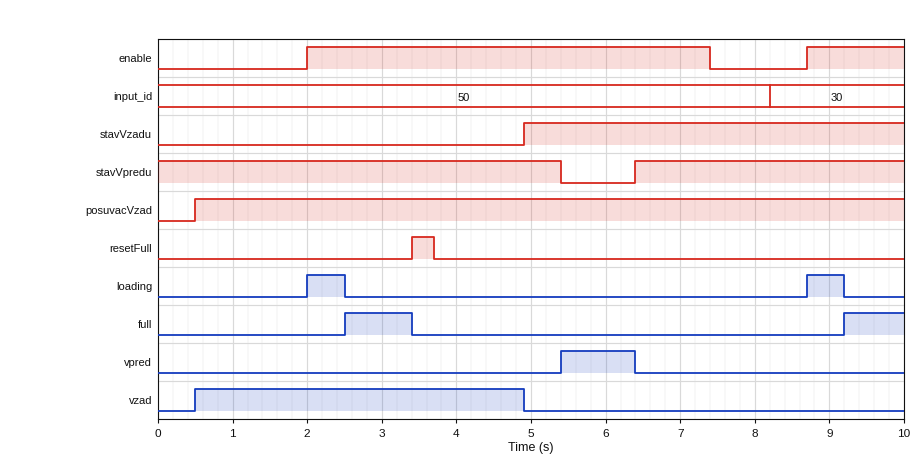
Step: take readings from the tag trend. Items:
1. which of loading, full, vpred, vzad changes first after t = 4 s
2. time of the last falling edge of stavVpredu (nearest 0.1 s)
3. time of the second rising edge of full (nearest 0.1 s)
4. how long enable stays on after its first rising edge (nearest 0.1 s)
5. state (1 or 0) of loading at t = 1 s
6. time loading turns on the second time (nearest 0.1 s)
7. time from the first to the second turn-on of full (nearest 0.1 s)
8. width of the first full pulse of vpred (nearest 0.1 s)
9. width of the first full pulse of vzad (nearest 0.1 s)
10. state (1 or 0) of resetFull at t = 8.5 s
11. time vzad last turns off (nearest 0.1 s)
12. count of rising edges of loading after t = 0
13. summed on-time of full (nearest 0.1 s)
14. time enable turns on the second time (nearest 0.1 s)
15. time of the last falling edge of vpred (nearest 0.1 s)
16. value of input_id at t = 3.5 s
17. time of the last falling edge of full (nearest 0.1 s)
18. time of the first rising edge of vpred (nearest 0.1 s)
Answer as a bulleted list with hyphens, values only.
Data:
- vzad
- 5.4 s
- 9.2 s
- 5.4 s
- 0
- 8.7 s
- 6.7 s
- 1.0 s
- 4.4 s
- 0
- 4.9 s
- 2
- 1.7 s
- 8.7 s
- 6.4 s
- 50
- 3.4 s
- 5.4 s
